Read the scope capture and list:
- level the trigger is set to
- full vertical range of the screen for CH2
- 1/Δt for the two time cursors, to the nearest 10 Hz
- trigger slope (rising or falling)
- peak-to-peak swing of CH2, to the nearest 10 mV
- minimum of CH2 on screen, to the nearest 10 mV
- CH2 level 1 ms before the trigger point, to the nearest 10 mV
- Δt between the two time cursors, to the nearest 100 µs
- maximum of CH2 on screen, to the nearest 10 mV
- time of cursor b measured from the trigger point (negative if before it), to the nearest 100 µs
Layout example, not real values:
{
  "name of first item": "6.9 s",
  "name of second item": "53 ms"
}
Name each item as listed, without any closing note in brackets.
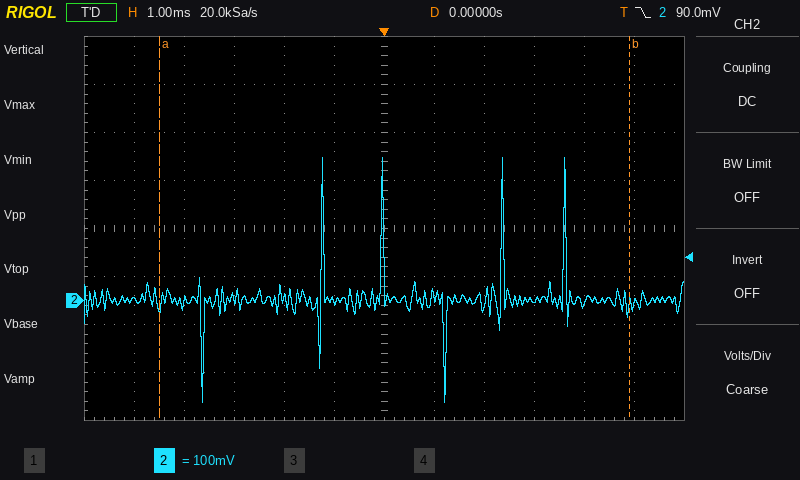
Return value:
{
  "level the trigger is set to": "90.0 mV",
  "full vertical range of the screen for CH2": "800 mV",
  "1/Δt for the two time cursors, to the nearest 10 Hz": "110 Hz",
  "trigger slope": "falling",
  "peak-to-peak swing of CH2, to the nearest 10 mV": "510 mV",
  "minimum of CH2 on screen, to the nearest 10 mV": "-210 mV",
  "CH2 level 1 ms before the trigger point, to the nearest 10 mV": "0 mV",
  "Δt between the two time cursors, to the nearest 100 µs": "9.4 ms",
  "maximum of CH2 on screen, to the nearest 10 mV": "300 mV",
  "time of cursor b measured from the trigger point (negative if before it), to the nearest 100 µs": "+4.9 ms"
}
